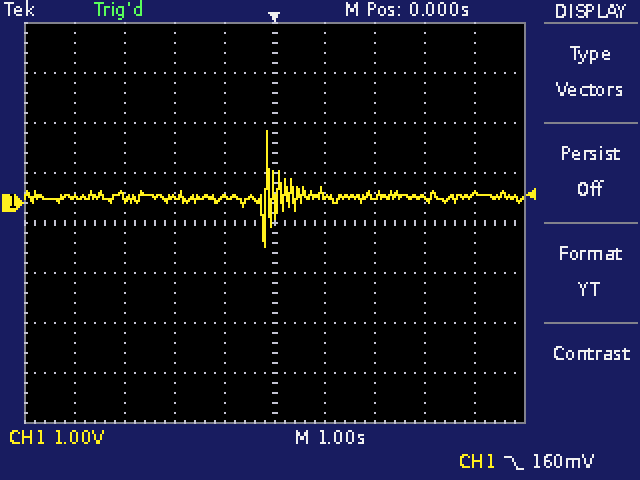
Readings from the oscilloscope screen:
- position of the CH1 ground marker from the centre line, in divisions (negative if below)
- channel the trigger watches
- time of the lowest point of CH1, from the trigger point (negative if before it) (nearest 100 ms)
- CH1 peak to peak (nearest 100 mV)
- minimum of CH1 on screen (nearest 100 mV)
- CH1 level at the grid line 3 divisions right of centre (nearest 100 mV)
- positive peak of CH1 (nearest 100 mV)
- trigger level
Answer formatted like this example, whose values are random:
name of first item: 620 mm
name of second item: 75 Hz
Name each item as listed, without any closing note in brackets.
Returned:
position of the CH1 ground marker from the centre line, in divisions: +0.4 div
channel the trigger watches: CH1
time of the lowest point of CH1, from the trigger point (negative if before it): -200 ms
CH1 peak to peak: 2.3 V
minimum of CH1 on screen: -900 mV
CH1 level at the grid line 3 divisions right of centre: 100 mV
positive peak of CH1: 1.4 V
trigger level: 160 mV
